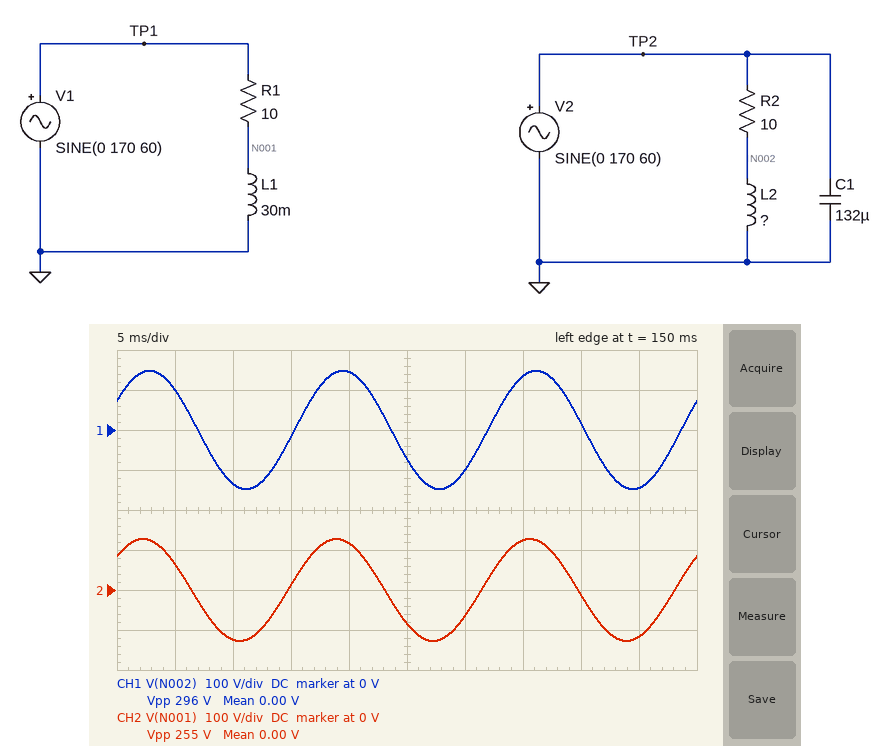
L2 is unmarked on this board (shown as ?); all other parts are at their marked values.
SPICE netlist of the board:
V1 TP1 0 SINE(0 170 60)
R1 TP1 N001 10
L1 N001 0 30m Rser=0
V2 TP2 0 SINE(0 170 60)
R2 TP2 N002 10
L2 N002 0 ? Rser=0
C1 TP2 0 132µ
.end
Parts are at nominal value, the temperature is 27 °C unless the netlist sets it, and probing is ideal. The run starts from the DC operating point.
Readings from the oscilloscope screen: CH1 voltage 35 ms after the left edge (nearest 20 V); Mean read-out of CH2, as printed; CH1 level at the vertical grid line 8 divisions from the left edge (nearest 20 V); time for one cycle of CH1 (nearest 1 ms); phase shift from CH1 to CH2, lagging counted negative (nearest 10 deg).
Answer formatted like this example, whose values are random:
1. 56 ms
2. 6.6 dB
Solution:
1. 140 V
2. 0.00 V
3. 20 V
4. 17 ms
5. 10 deg
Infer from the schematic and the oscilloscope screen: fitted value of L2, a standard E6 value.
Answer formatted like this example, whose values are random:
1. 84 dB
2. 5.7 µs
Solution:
1. 47 mH
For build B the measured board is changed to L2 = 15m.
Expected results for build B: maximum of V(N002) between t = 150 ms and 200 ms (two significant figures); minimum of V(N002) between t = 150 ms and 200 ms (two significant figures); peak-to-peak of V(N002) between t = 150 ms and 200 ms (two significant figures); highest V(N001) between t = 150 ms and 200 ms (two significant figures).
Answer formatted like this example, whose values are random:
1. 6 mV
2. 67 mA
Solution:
1. 84 V
2. -84 V
3. 170 V
4. 130 V
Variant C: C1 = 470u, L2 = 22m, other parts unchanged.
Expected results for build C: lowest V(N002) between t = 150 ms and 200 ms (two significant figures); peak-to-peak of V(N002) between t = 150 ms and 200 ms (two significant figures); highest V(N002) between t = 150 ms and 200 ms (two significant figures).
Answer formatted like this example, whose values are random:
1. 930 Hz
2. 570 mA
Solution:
1. -110 V
2. 220 V
3. 110 V
